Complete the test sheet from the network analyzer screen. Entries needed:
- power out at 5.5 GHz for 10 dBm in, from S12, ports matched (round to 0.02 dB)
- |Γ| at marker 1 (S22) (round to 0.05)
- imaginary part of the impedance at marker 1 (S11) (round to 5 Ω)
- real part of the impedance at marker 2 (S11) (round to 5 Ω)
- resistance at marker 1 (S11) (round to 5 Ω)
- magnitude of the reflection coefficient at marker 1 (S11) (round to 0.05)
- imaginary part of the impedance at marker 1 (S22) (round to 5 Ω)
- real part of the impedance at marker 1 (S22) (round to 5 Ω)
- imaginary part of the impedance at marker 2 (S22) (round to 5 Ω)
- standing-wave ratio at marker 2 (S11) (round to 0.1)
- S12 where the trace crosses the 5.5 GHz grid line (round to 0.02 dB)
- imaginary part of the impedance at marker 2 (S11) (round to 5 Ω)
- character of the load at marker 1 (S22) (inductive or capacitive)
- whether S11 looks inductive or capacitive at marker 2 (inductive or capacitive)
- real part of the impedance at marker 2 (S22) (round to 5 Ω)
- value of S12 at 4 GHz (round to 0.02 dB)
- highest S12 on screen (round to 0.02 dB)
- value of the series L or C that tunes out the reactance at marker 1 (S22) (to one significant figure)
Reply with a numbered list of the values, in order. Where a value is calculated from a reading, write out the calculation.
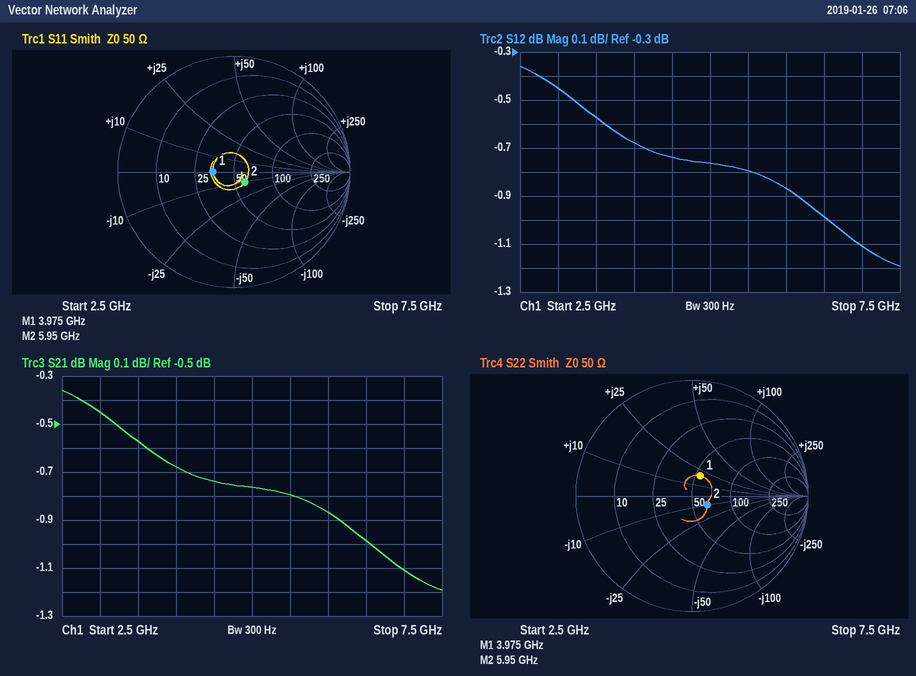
1. 10 dBm + (-0.80 dB) = 9.20 dBm
2. 0.20
3. 0 Ω
4. 60 Ω
5. 35 Ω
6. 0.20
7. +20 Ω
8. 55 Ω
9. -10 Ω
10. 1.3
11. -0.80 dB
12. -10 Ω
13. inductive
14. capacitive
15. 65 Ω
16. -0.68 dB
17. -0.36 dB
18. C = 1/(2π × 3.975 GHz × 20 Ω) ≈ 2 pF
